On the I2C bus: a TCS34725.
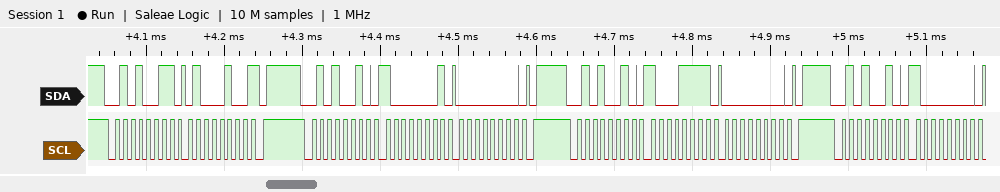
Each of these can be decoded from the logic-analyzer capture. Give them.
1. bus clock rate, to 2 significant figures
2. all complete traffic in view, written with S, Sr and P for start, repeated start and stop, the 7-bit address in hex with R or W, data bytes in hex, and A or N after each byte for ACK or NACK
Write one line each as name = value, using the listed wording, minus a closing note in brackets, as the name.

bus clock rate, to 2 significant figures = 100 kHz
all complete traffic in view, written with S, Sr and P for start, repeated start and stop, the 7-bit address in hex with R or W, data bytes in hex, and A or N after each byte for ACK or NACK = S 29R A 44 N P S 29W A 81 A 00 A P S 29W A 8F A 00 A P S 29W A 80 A
